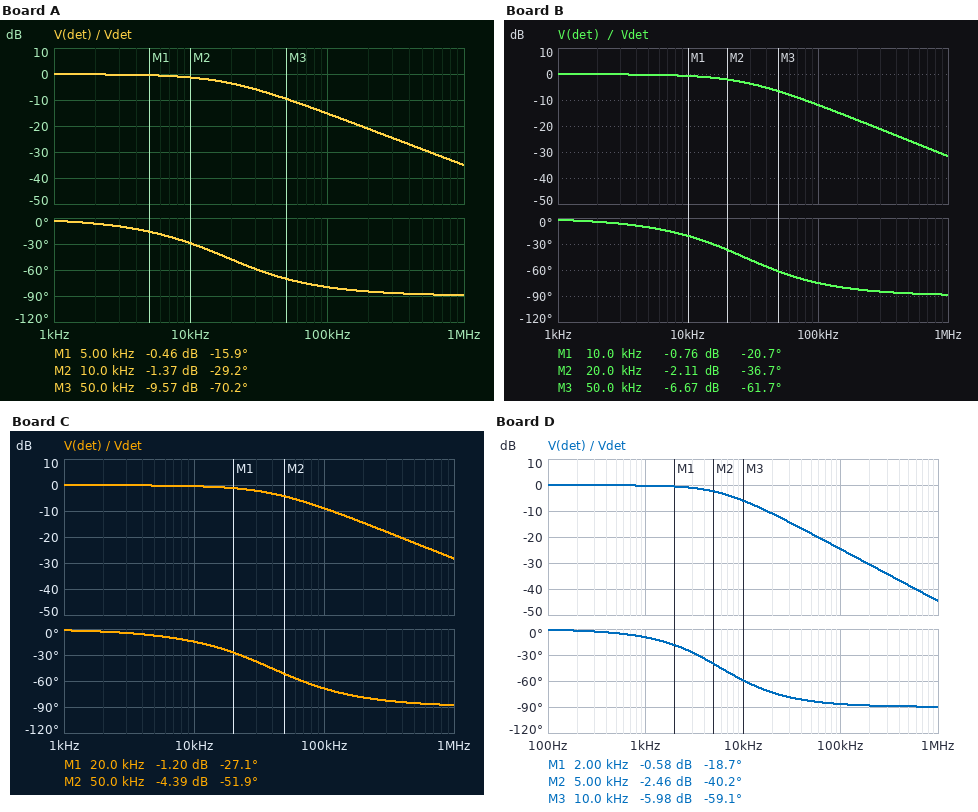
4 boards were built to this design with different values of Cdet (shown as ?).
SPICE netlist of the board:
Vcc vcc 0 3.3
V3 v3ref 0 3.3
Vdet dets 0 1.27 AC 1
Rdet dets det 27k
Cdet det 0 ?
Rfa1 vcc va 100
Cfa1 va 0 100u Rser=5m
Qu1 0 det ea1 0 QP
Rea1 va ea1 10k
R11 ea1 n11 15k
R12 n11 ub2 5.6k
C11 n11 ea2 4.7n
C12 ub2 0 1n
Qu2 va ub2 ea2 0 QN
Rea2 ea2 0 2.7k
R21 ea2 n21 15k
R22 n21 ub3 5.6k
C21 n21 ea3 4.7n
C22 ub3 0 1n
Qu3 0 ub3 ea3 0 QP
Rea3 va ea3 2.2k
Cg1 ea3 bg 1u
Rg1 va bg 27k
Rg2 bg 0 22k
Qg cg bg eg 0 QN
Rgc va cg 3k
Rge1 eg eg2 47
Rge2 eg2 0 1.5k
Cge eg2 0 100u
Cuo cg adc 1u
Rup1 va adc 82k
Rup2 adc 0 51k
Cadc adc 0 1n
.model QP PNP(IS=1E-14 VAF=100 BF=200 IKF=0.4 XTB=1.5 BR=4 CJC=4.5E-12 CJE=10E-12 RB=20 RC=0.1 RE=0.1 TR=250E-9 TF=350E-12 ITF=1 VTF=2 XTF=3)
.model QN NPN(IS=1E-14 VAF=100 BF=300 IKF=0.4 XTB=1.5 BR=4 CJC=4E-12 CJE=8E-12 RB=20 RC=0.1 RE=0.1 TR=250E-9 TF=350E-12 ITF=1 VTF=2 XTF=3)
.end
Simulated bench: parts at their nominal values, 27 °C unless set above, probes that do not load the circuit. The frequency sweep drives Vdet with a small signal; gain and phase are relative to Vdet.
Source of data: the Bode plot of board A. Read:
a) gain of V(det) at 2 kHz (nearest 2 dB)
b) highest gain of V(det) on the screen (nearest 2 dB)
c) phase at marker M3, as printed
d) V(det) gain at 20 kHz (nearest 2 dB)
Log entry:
0 dB
0 dB
-70.2 deg
-4 dB
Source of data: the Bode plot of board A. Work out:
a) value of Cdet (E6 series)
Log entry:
330 pF
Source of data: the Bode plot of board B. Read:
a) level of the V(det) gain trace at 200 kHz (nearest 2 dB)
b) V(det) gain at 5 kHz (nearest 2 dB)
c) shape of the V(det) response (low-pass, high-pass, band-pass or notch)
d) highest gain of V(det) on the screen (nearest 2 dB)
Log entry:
-18 dB
0 dB
low-pass
0 dB
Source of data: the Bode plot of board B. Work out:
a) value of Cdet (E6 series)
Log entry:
220 pF
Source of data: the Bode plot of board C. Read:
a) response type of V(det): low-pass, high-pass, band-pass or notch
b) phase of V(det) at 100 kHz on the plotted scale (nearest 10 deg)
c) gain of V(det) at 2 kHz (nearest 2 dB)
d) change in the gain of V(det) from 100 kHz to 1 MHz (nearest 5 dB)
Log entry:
low-pass
-70 deg
0 dB
-20 dB
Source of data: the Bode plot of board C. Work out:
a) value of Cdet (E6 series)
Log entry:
150 pF
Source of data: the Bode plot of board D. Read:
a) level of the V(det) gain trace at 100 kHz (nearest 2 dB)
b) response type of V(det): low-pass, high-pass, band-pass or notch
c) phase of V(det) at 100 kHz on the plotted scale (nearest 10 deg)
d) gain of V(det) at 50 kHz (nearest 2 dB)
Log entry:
-24 dB
low-pass
-90 deg
-18 dB
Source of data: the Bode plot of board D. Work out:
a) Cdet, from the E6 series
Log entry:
1 nF
